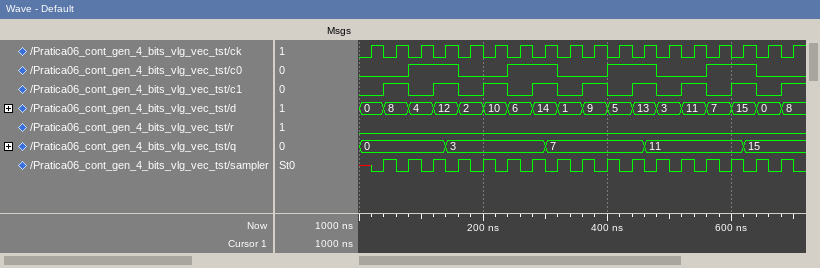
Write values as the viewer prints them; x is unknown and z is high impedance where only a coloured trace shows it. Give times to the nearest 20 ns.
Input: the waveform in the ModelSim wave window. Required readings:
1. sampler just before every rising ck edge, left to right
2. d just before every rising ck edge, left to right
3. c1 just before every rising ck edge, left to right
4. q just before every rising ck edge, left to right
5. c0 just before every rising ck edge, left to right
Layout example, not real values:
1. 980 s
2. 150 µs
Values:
1. x 1 1 1 1 1 1 1 1 1 1 1 1 1 1 1 1 1
2. 0, 8, 4, 12, 2, 10, 6, 14, 1, 9, 5, 13, 3, 11, 7, 15, 0, 8
3. 0 1 0 1 0 1 0 1 0 1 0 1 0 1 0 1 0 1
4. 0, 0, 0, 0, 3, 3, 3, 3, 7, 7, 7, 7, 11, 11, 11, 11, 15, 15
5. 0 0 1 1 0 0 1 1 0 0 1 1 0 0 1 1 0 0
